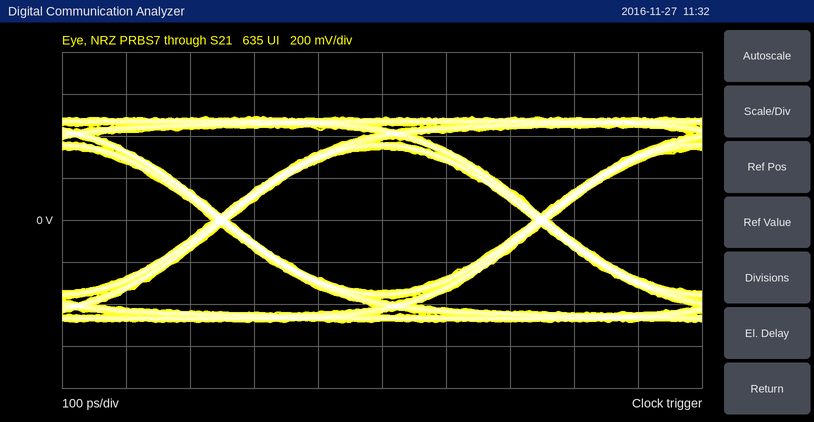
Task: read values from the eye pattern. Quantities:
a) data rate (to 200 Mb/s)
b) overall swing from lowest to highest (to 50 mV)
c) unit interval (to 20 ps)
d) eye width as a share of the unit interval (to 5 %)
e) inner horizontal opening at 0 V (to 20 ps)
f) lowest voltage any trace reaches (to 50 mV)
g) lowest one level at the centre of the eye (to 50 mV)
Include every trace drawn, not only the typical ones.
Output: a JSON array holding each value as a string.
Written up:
["2.0 Gb/s", "1.00 V", "500 ps", "95 %", "480 ps", "-500 mV", "350 mV"]
